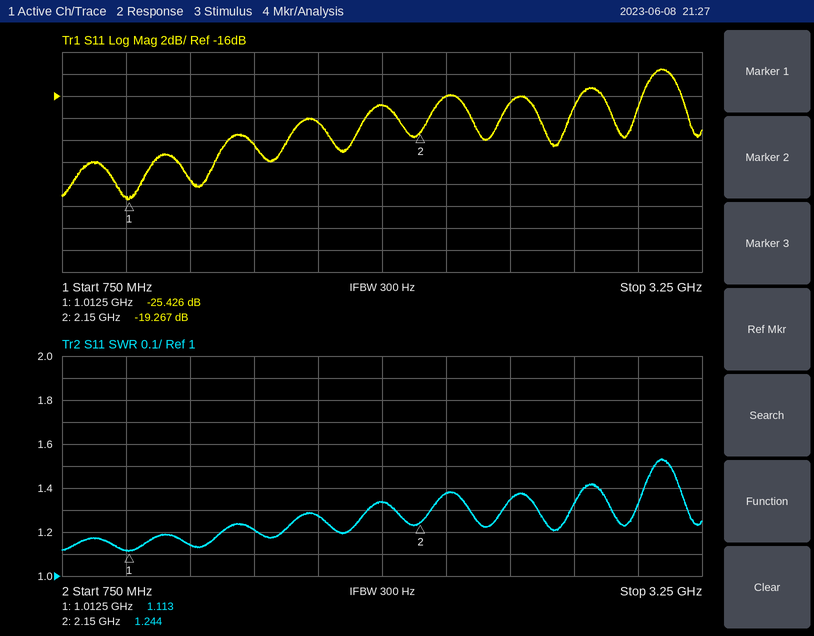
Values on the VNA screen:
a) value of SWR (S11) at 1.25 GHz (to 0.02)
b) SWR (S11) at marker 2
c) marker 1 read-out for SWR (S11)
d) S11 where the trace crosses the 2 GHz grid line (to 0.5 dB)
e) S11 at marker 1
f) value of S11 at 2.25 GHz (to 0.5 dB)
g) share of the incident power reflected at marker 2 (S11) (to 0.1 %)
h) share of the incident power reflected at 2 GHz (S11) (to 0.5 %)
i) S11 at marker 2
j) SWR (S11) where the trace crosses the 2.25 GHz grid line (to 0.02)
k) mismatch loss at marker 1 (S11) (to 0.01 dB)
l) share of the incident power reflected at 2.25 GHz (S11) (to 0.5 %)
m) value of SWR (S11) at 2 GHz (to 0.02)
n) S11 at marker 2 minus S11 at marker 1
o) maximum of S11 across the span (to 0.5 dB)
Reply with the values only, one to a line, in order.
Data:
1.14
1.244
1.113
-17.0 dB
-25.426 dB
-16.0 dB
1.2 %
2.0 %
-19.267 dB
1.38
0.01 dB
2.5 %
1.34
6.159 dB
-13.5 dB
